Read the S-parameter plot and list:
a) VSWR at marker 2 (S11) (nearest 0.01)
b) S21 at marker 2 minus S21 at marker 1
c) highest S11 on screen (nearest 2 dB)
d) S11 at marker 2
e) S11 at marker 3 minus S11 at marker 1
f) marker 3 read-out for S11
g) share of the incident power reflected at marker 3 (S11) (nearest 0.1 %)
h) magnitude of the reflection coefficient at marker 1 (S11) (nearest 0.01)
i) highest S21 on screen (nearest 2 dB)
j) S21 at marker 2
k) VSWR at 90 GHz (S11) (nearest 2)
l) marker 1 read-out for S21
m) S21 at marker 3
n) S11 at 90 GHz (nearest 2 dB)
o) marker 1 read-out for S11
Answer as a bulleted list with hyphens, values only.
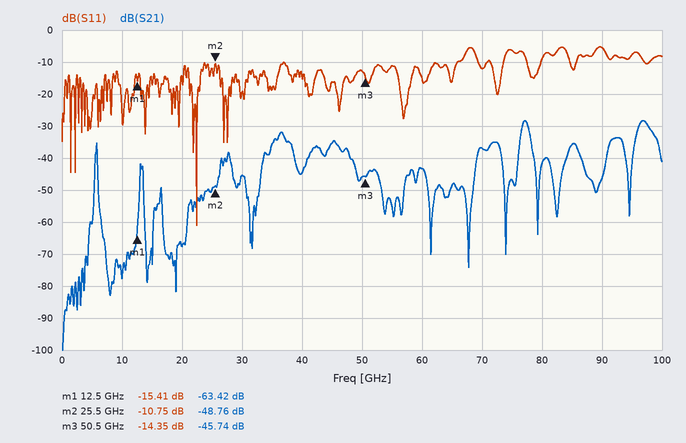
- 1.82
- 14.66 dB
- -6 dB
- -10.75 dB
- 1.06 dB
- -14.35 dB
- 3.7 %
- 0.17
- -28 dB
- -48.76 dB
- 4
- -63.42 dB
- -45.74 dB
- -6 dB
- -15.41 dB
